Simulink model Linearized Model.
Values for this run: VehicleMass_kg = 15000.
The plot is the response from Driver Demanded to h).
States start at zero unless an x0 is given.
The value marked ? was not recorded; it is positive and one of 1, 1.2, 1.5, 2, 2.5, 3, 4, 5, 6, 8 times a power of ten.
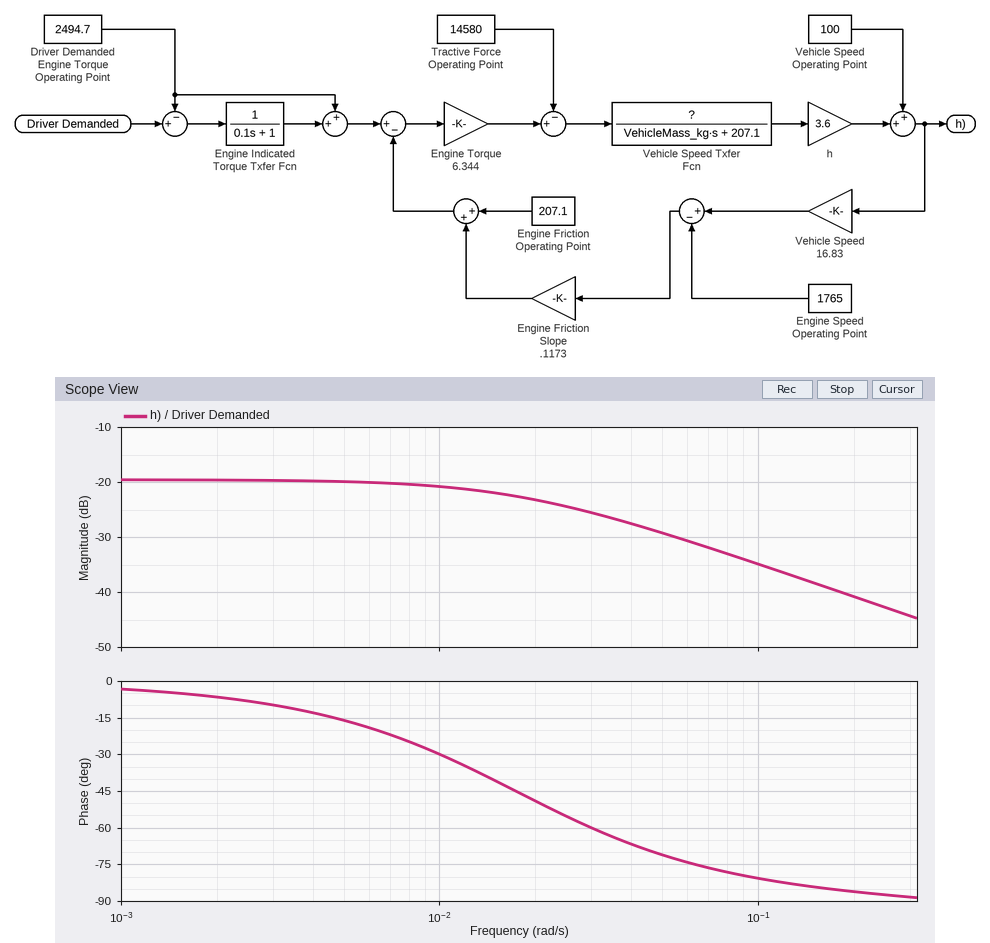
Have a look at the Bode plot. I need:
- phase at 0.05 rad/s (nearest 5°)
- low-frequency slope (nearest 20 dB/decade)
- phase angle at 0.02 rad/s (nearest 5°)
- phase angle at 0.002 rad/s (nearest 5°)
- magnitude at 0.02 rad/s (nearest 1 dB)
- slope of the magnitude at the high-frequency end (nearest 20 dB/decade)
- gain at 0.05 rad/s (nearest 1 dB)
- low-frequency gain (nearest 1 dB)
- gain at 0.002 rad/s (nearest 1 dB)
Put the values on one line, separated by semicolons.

-70°; 0 dB/decade; -50°; -5°; -23 dB; -20 dB/decade; -29 dB; -20 dB; -20 dB
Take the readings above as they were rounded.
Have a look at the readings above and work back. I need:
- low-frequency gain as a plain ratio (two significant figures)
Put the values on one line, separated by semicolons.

0.10
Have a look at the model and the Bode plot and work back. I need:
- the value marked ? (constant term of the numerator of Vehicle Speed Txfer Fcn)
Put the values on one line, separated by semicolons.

1.2
